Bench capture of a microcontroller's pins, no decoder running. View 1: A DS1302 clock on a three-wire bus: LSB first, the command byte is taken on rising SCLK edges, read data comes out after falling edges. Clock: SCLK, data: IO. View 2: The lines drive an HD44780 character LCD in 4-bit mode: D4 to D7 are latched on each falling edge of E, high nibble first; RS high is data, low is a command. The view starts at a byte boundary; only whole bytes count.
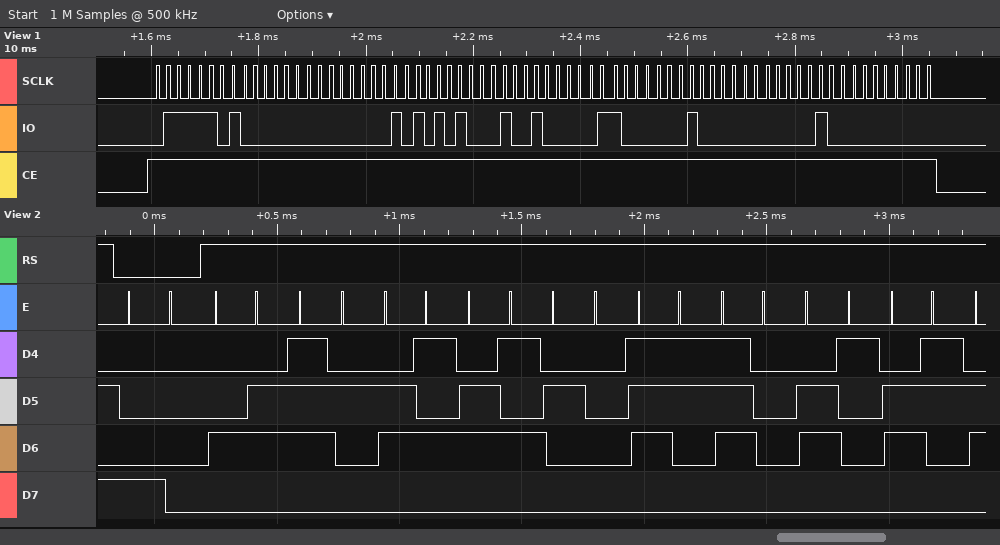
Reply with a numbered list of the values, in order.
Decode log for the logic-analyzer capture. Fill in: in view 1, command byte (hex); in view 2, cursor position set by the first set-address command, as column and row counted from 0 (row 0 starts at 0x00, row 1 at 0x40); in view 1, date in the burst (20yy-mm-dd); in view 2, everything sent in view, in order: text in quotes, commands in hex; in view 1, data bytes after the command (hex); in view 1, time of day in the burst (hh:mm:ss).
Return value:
1. 0xBE
2. column 0, row 0
3. 2020-06-09
4. 0x80 "Free spac"
5. 00 40 15 09 06 02 20 00
6. 15:40:00
